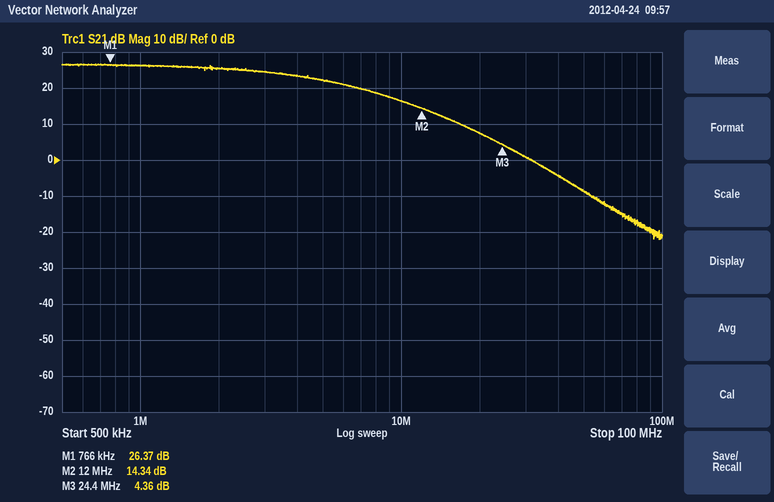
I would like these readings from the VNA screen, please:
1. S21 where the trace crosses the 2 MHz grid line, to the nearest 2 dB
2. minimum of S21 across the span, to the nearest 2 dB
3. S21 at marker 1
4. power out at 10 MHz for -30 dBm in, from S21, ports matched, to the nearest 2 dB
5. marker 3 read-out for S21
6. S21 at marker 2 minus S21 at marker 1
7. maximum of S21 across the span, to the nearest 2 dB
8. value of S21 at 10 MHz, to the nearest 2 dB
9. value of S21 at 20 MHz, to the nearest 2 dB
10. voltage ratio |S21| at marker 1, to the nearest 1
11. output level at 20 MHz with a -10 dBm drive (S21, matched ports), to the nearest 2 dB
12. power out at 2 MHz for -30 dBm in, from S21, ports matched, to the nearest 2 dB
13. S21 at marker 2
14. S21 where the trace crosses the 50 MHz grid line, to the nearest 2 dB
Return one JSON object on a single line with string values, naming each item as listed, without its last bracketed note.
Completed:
{"S21 where the trace crosses the 2 MHz grid line, to the nearest 2 dB": "26 dB", "minimum of S21 across the span, to the nearest 2 dB": "-22 dB", "S21 at marker 1": "26.37 dB", "power out at 10 MHz for -30 dBm in, from S21, ports matched, to the nearest 2 dB": "-14 dBm", "marker 3 read-out for S21": "4.36 dB", "S21 at marker 2 minus S21 at marker 1": "-12.03 dB", "maximum of S21 across the span, to the nearest 2 dB": "26 dB", "value of S21 at 10 MHz, to the nearest 2 dB": "16 dB", "value of S21 at 20 MHz, to the nearest 2 dB": "8 dB", "voltage ratio |S21| at marker 1, to the nearest 1": "21", "output level at 20 MHz with a -10 dBm drive (S21, matched ports), to the nearest 2 dB": "-2 dBm", "power out at 2 MHz for -30 dBm in, from S21, ports matched, to the nearest 2 dB": "-4 dBm", "S21 at marker 2": "14.34 dB", "S21 where the trace crosses the 50 MHz grid line, to the nearest 2 dB": "-8 dB"}
